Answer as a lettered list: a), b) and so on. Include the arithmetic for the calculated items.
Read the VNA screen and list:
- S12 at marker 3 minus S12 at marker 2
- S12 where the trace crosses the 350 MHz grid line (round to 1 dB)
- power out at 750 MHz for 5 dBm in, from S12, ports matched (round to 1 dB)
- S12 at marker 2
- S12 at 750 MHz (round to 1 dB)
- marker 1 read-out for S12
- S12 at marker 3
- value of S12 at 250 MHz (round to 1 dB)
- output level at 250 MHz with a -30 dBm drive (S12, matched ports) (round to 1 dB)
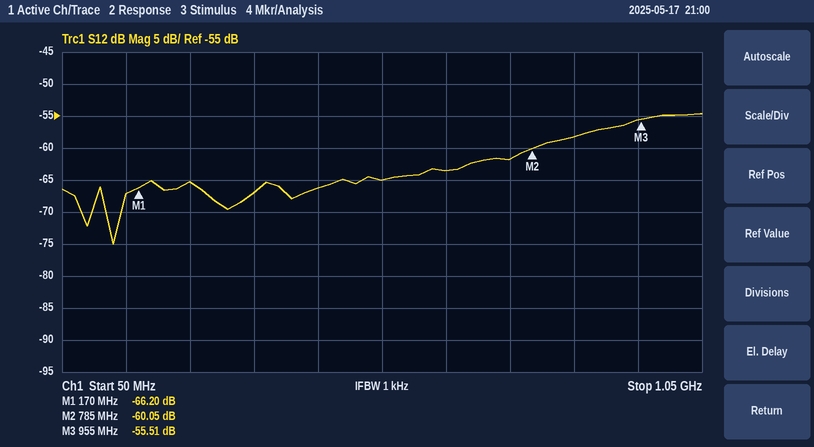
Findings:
a) -55.51 − (-60.05) = 4.54 dB
b) -67 dB
c) 5 dBm + (-62 dB) = -57 dBm
d) -60.05 dB
e) -62 dB
f) -66.20 dB
g) -55.51 dB
h) -65 dB
i) -30 dBm + (-65 dB) = -95 dBm
